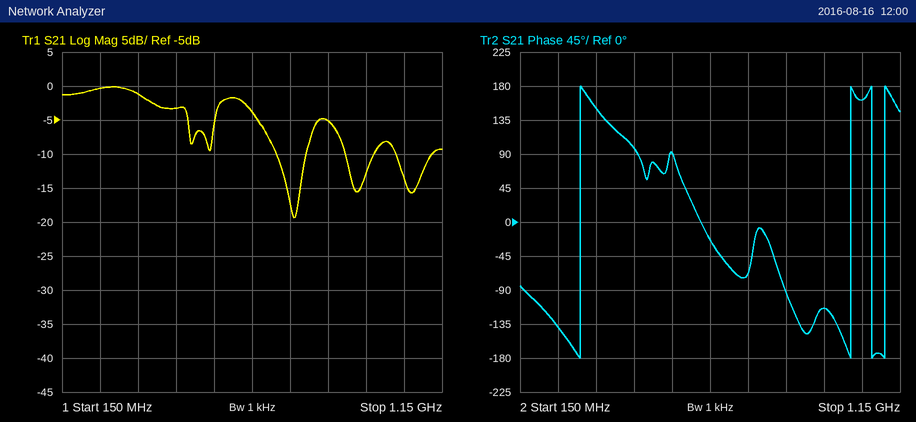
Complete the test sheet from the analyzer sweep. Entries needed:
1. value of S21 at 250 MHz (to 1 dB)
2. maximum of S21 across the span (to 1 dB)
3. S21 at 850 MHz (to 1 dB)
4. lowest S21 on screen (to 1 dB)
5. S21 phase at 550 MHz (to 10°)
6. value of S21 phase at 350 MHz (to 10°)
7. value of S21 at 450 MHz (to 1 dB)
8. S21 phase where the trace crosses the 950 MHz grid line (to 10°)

0 dB
0 dB
-5 dB
-19 dB
90°
150°
-3 dB
-110°
